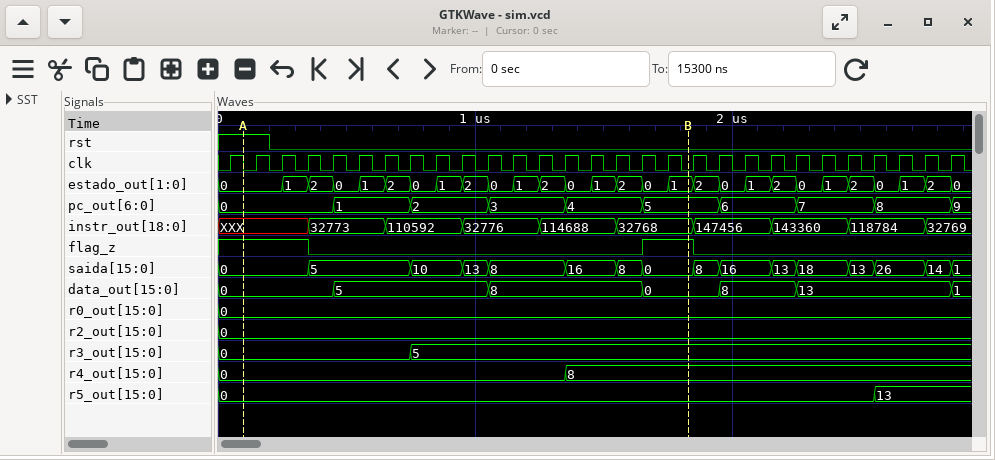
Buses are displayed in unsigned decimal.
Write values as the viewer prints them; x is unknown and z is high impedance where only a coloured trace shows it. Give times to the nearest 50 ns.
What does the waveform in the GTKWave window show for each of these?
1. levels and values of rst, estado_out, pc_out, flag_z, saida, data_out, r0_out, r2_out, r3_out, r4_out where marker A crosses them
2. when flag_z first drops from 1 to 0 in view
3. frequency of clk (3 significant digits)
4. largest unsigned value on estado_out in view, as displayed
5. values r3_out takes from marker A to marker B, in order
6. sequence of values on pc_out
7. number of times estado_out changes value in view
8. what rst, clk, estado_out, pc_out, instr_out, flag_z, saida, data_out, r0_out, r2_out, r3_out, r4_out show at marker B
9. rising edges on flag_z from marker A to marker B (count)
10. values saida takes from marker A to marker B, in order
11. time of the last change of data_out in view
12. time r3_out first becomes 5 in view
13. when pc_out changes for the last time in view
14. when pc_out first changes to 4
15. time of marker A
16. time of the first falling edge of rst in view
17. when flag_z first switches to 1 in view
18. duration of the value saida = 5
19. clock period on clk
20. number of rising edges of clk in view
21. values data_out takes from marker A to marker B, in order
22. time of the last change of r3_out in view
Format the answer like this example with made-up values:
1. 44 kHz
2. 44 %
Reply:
1. rst=1, estado_out=0, pc_out=0, flag_z=1, saida=0, data_out=0, r0_out=0, r2_out=0, r3_out=0, r4_out=0
2. 350 ns
3. 10.0 MHz
4. 2
5. 0, 5
6. 0, 1, 2, 3, 4, 5, 6, 7, 8, 9
7. 27
8. rst=0, clk=0, estado_out=1, pc_out=5, instr_out=32768, flag_z=1, saida=0, data_out=0, r0_out=0, r2_out=0, r3_out=5, r4_out=8
9. 1
10. 0, 5, 10, 13, 8, 16, 8, 0
11. 2850 ns
12. 750 ns
13. 2850 ns
14. 1350 ns
15. 100 ns
16. 200 ns
17. 1650 ns
18. 400 ns
19. 100 ns
20. 29
21. 0, 5, 8, 0
22. 750 ns
